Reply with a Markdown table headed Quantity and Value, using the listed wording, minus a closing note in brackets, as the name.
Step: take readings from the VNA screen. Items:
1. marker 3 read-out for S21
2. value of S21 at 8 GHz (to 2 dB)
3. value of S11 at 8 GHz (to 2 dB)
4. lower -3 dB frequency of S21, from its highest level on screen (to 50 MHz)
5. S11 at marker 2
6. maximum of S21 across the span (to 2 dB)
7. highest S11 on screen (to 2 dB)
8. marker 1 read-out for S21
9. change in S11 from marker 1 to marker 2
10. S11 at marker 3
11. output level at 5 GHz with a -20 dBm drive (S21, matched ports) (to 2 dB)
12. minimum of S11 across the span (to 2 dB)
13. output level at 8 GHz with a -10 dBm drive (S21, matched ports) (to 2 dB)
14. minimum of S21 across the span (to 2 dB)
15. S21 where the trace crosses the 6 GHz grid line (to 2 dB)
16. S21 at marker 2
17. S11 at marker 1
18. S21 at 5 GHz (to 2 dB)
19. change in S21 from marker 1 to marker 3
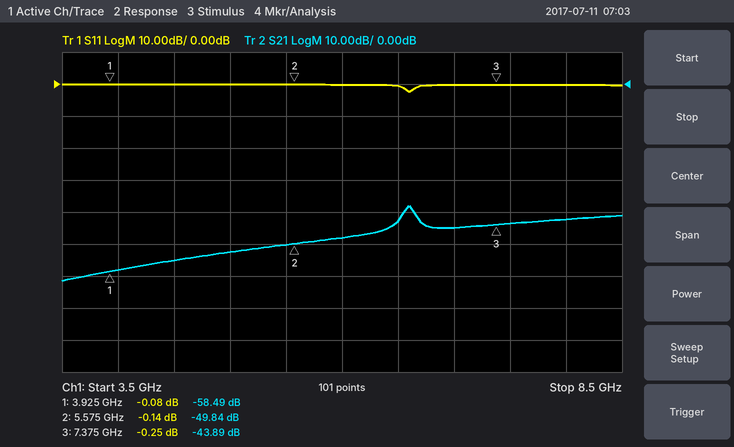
| Quantity | Value |
|---|---|
| marker 3 read-out for S21 | -43.89 dB |
| value of S21 at 8 GHz | -42 dB |
| value of S11 at 8 GHz | 0 dB |
| lower -3 dB frequency of S21, from its highest level on screen | 6.55 GHz |
| S11 at marker 2 | -0.14 dB |
| maximum of S21 across the span | -38 dB |
| highest S11 on screen | 0 dB |
| marker 1 read-out for S21 | -58.49 dB |
| change in S11 from marker 1 to marker 2 | -0.06 dB |
| S11 at marker 3 | -0.25 dB |
| output level at 5 GHz with a -20 dBm drive (S21, matched ports) | -72 dBm |
| minimum of S11 across the span | -2 dB |
| output level at 8 GHz with a -10 dBm drive (S21, matched ports) | -52 dBm |
| minimum of S21 across the span | -62 dB |
| S21 where the trace crosses the 6 GHz grid line | -48 dB |
| S21 at marker 2 | -49.84 dB |
| S11 at marker 1 | -0.08 dB |
| S21 at 5 GHz | -52 dB |
| change in S21 from marker 1 to marker 3 | 14.60 dB |
